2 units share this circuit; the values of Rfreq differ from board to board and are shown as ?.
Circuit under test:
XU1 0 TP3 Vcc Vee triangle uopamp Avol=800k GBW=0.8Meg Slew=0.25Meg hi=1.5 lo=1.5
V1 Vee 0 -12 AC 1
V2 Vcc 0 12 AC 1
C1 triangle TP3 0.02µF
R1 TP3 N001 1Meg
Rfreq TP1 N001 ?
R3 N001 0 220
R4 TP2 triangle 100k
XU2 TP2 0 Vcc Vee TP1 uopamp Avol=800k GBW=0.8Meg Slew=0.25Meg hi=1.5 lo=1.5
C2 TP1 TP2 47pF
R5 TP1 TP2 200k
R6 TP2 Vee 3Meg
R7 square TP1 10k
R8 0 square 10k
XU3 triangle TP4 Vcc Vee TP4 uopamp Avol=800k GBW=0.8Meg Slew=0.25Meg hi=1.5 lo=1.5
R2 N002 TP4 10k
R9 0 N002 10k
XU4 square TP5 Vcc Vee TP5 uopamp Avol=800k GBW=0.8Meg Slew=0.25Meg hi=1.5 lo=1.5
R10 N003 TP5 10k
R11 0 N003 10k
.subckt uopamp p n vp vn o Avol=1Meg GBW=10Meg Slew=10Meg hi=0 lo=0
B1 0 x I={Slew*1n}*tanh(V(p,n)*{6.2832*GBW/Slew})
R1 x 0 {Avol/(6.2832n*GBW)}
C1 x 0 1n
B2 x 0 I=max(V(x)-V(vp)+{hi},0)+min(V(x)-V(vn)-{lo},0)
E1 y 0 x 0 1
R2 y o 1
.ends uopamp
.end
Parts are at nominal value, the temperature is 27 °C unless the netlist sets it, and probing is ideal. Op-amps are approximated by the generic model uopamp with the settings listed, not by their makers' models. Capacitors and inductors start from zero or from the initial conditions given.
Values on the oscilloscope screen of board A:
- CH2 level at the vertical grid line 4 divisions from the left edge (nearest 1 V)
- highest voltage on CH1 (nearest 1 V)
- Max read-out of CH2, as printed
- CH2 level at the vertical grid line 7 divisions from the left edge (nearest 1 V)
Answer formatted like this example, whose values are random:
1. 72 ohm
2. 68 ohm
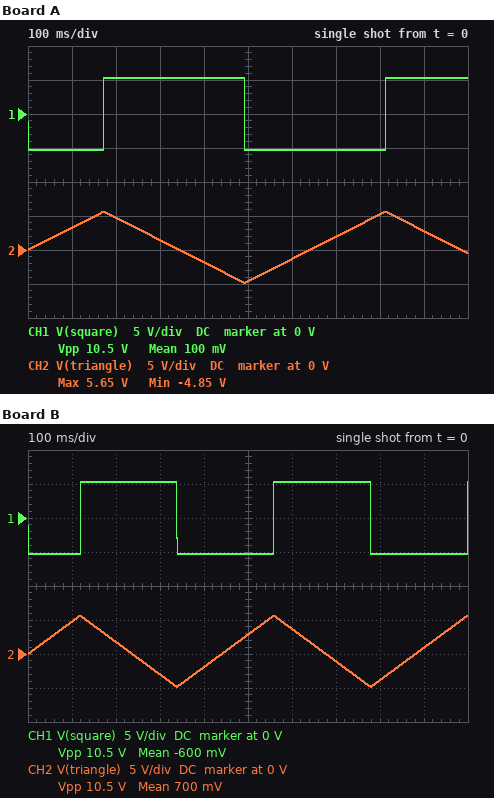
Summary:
1. -2 V
2. 5 V
3. 5.65 V
4. 2 V
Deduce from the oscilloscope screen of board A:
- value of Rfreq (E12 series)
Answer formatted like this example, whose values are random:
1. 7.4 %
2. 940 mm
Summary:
1. 3.3 kΩ
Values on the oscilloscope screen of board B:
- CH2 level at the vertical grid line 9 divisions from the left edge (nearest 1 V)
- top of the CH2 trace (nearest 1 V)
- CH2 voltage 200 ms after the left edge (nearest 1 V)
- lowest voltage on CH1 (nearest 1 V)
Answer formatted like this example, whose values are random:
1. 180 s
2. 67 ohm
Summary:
1. 1 V
2. 6 V
3. 2 V
4. -5 V
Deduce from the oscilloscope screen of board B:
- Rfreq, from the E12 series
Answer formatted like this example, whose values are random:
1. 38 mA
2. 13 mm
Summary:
1. 2.2 kΩ
